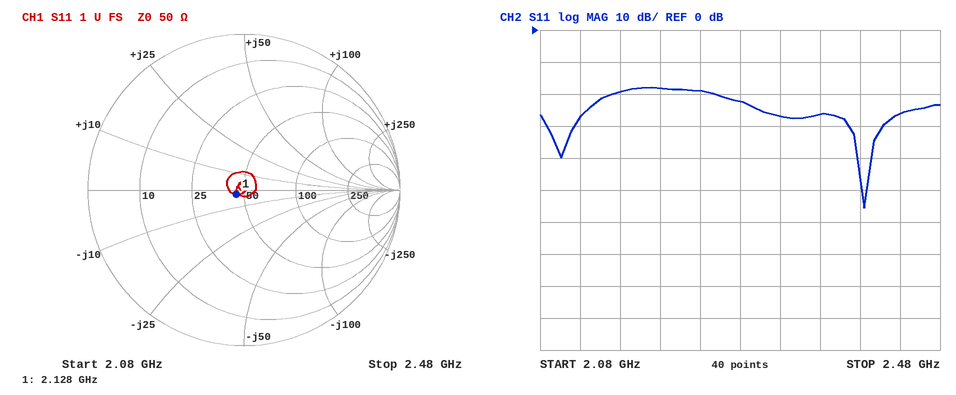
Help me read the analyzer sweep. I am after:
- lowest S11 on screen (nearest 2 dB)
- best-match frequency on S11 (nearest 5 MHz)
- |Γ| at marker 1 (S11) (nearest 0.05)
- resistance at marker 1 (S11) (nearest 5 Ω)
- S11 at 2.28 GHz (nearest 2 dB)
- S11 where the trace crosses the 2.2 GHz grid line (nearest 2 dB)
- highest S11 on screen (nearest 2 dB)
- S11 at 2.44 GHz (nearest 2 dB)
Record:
-56 dB
2.405 GHz
0.05
45 Ω
-22 dB
-18 dB
-18 dB
-26 dB
